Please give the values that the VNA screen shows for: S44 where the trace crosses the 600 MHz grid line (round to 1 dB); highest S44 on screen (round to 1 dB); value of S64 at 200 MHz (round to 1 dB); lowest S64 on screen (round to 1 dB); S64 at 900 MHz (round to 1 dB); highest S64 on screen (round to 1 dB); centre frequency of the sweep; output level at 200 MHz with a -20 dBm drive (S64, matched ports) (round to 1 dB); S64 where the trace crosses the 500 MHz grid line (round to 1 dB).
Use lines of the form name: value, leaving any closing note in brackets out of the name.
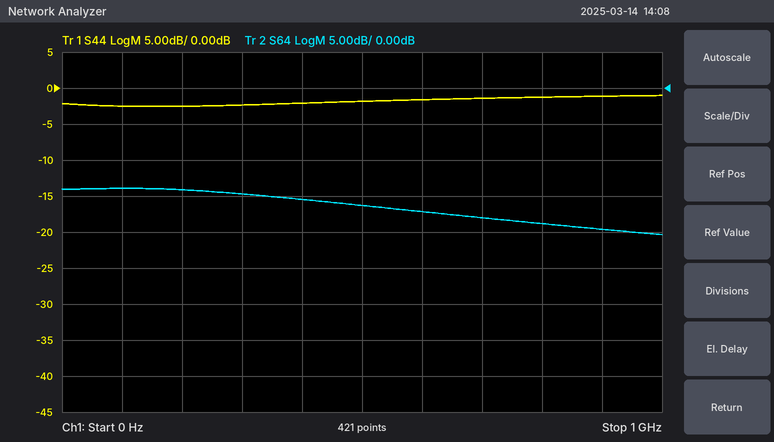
S44 where the trace crosses the 600 MHz grid line: -2 dB
highest S44 on screen: -1 dB
value of S64 at 200 MHz: -14 dB
lowest S64 on screen: -20 dB
S64 at 900 MHz: -20 dB
highest S64 on screen: -14 dB
centre frequency of the sweep: 500 MHz
output level at 200 MHz with a -20 dBm drive (S64, matched ports): -34 dBm
S64 where the trace crosses the 500 MHz grid line: -16 dB
